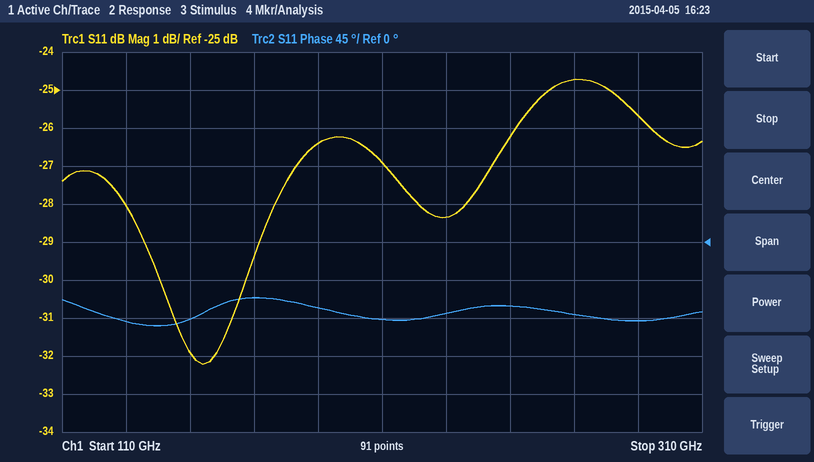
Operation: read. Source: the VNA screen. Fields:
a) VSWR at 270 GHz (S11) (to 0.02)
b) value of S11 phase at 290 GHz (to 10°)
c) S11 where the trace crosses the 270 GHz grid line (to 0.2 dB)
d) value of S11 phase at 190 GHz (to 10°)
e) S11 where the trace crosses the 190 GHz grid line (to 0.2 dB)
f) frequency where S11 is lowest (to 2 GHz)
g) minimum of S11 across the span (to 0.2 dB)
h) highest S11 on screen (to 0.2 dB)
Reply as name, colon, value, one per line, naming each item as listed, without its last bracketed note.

VSWR at 270 GHz (S11): 1.12
value of S11 phase at 290 GHz: -90°
S11 where the trace crosses the 270 GHz grid line: -24.8 dB
value of S11 phase at 190 GHz: -80°
S11 where the trace crosses the 190 GHz grid line: -26.4 dB
frequency where S11 is lowest: 154 GHz
minimum of S11 across the span: -32.2 dB
highest S11 on screen: -24.8 dB
